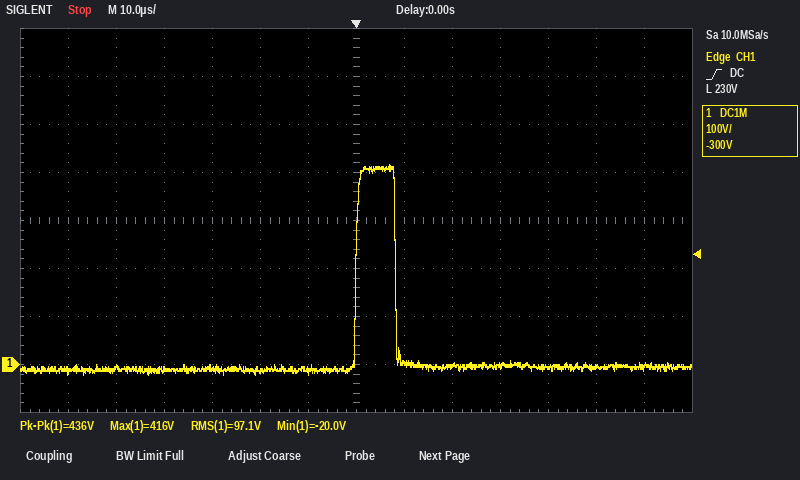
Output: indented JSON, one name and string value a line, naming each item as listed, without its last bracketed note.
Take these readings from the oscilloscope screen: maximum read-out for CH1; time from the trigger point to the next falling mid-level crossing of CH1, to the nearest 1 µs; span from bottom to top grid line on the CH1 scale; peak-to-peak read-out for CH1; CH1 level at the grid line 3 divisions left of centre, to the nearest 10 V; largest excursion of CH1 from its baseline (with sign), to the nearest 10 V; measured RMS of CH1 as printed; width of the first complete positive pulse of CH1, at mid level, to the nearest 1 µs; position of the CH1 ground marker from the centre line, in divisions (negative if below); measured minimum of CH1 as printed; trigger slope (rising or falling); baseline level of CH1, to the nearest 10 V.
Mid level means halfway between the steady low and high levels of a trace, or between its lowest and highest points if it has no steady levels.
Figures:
{
  "maximum read-out for CH1": "416 V",
  "time from the trigger point to the next falling mid-level crossing of CH1, to the nearest 1 µs": "8 µs",
  "span from bottom to top grid line on the CH1 scale": "800 V",
  "peak-to-peak read-out for CH1": "436 V",
  "CH1 level at the grid line 3 divisions left of centre, to the nearest 10 V": "-10 V",
  "largest excursion of CH1 from its baseline (with sign), to the nearest 10 V": "+420 V",
  "measured RMS of CH1 as printed": "97.1 V",
  "width of the first complete positive pulse of CH1, at mid level, to the nearest 1 µs": "8 µs",
  "position of the CH1 ground marker from the centre line, in divisions": "-3.0 div",
  "measured minimum of CH1 as printed": "-20.0 V",
  "trigger slope": "rising",
  "baseline level of CH1, to the nearest 10 V": "-10 V"
}
